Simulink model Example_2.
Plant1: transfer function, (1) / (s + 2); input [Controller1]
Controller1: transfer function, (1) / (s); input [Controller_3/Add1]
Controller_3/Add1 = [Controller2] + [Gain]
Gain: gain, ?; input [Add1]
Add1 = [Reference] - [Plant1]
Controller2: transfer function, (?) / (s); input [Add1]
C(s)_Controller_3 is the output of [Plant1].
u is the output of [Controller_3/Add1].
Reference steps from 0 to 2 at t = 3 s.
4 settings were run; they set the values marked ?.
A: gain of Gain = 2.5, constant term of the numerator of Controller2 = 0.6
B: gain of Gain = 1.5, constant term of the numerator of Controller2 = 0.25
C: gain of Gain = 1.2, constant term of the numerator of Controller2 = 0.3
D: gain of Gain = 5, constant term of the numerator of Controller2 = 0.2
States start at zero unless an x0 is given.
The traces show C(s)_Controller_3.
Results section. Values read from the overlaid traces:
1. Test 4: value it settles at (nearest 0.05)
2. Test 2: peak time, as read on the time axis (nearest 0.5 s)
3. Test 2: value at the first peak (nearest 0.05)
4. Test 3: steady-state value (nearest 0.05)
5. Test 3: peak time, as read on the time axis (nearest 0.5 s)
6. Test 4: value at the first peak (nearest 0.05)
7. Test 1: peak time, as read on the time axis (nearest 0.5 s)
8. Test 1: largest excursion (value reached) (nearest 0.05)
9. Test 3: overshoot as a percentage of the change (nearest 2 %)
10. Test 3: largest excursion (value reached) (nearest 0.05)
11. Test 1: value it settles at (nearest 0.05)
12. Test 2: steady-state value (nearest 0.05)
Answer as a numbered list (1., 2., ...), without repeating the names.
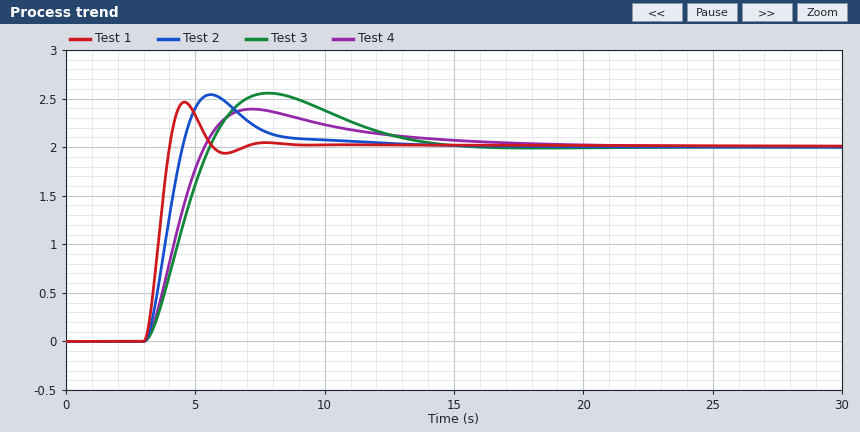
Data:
1. 2.00
2. 5.5 s
3. 2.55
4. 2.00
5. 8.0 s
6. 2.40
7. 4.5 s
8. 2.45
9. 28 %
10. 2.55
11. 2.00
12. 2.00
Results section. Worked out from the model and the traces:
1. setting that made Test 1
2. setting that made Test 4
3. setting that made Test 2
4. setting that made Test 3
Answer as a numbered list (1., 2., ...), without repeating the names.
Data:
1. D
2. B
3. A
4. C
